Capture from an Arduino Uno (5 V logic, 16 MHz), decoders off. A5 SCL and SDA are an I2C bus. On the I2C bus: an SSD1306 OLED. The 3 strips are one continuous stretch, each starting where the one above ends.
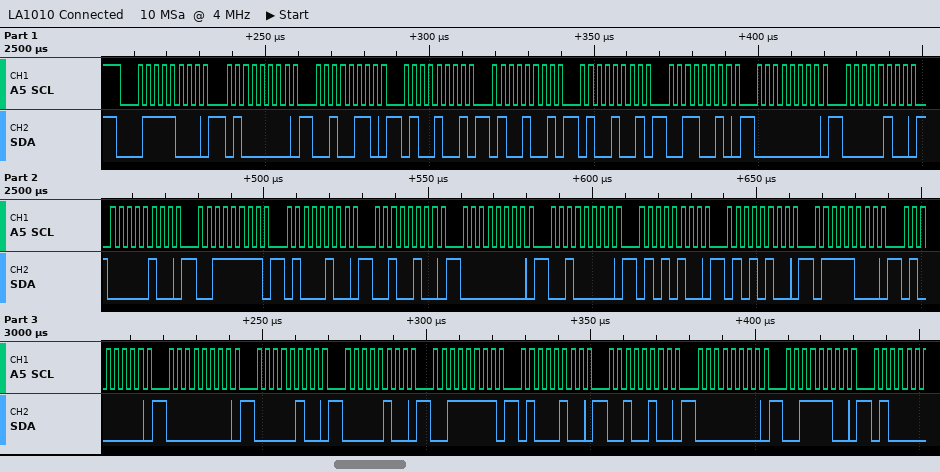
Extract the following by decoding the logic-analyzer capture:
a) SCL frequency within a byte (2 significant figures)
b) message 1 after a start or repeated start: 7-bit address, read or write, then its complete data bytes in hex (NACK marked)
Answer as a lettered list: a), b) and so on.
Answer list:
a) 400 kHz
b) 0x3C write: 40 26 49 49 49 32 00 04 04 3F 44 24 00 20 54 54 78 40 00 04 04 3F 44 24 00 3C
